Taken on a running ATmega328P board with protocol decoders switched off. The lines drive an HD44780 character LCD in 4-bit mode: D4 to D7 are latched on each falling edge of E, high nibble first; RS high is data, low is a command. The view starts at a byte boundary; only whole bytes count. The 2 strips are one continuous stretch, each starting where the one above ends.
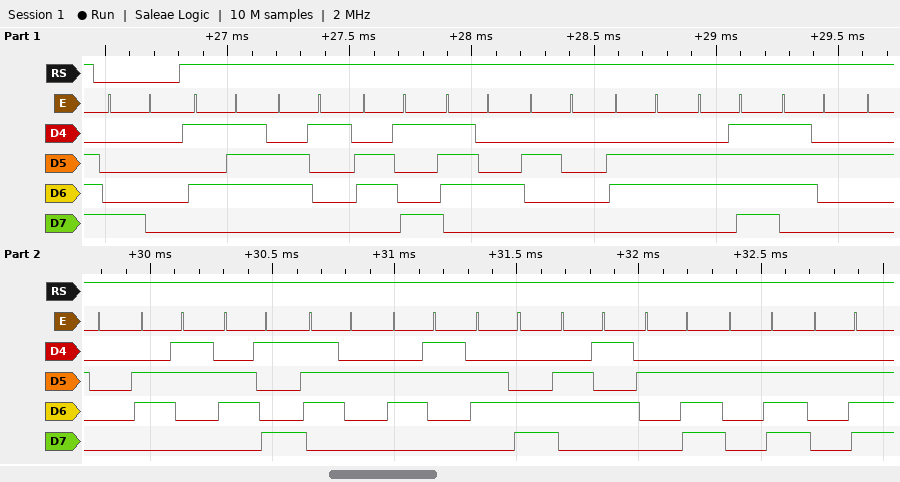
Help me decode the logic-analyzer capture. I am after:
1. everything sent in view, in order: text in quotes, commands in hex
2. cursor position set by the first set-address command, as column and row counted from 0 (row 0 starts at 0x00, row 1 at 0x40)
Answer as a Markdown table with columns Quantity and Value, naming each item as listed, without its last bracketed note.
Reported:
| Quantity | Value |
|---|---|
| everything sent in view, in order: text in quotes, commands in hex | 0x80 "Wait for circle..." |
| cursor position set by the first set-address command, as column and row counted from 0 | column 0, row 0 |
